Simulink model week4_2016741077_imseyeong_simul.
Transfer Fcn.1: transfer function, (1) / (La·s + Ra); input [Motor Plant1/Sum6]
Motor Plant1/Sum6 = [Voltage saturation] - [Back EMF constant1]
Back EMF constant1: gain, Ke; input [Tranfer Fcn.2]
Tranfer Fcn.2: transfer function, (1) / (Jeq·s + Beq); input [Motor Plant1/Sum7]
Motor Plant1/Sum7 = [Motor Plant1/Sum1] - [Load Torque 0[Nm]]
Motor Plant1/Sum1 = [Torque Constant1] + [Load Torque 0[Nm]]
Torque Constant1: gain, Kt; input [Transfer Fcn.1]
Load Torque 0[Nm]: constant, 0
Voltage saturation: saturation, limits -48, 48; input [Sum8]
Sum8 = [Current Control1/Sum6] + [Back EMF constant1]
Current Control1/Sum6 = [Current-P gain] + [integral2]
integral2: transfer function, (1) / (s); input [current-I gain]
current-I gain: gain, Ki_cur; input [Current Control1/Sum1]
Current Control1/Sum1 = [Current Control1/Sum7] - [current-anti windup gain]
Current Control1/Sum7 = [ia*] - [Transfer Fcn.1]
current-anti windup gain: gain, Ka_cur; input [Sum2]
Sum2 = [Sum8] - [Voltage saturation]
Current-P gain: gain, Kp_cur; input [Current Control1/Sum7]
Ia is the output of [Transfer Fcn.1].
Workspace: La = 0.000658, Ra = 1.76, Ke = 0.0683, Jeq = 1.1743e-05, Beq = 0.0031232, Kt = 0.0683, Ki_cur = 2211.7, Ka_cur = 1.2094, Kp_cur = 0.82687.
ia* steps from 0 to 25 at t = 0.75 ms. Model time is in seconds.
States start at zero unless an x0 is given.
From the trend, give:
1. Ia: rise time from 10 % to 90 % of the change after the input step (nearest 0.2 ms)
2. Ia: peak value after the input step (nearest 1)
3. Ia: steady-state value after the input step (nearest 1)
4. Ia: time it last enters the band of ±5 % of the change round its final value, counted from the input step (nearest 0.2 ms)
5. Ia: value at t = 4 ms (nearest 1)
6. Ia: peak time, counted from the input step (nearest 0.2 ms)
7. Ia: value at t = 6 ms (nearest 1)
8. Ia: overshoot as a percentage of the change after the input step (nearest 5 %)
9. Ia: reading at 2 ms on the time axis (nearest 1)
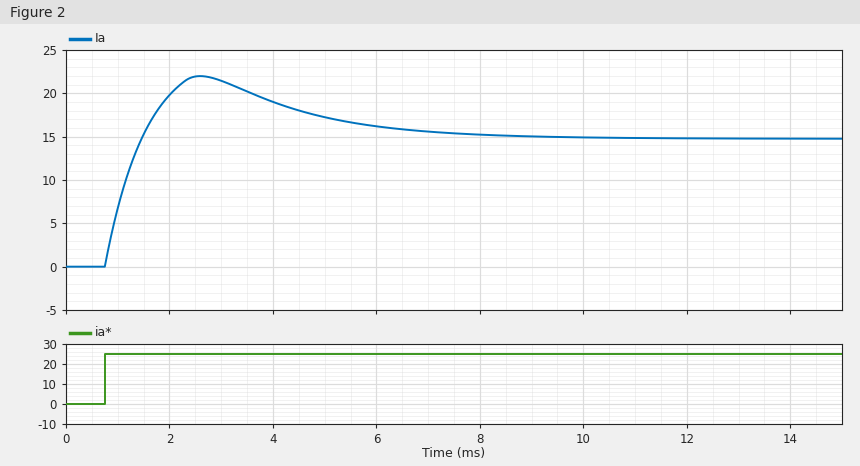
0.6 ms
22
15
6.4 ms
19
1.8 ms
16
50 %
20
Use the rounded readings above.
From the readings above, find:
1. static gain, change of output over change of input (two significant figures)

0.60
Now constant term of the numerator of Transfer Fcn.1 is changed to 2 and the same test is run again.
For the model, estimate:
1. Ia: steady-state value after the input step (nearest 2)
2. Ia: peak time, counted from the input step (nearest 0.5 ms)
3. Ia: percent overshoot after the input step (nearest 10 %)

20
5.0 ms
20 %
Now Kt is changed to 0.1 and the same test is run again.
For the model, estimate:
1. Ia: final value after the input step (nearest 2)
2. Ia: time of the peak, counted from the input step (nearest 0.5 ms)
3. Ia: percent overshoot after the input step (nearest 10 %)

12
1.5 ms
70 %
